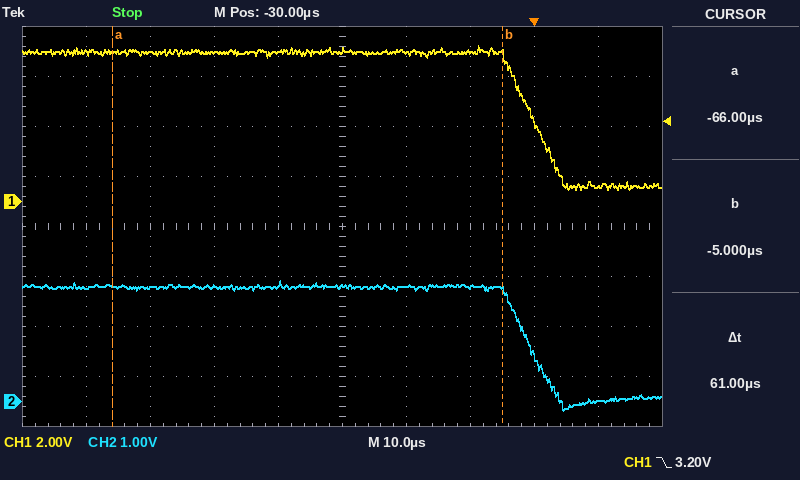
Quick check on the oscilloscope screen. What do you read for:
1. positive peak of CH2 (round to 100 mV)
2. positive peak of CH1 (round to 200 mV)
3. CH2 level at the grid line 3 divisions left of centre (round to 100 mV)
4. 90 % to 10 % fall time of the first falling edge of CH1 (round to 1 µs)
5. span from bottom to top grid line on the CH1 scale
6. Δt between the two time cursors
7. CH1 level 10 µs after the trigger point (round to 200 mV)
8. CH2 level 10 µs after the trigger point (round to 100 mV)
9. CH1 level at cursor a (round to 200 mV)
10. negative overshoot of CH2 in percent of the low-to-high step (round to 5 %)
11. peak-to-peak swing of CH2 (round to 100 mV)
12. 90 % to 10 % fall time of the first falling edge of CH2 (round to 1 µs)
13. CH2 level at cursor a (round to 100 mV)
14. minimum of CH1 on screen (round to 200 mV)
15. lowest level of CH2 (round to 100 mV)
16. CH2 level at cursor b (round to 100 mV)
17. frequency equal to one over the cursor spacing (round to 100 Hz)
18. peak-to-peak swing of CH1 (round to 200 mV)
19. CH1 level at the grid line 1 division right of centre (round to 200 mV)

2.4 V
6.2 V
2.3 V
8 µs
16 V
61 µs
600 mV
0.0 V
6.0 V
10 %
2.6 V
7 µs
2.3 V
400 mV
-200 mV
2.2 V
16.4 kHz
5.8 V
6.0 V
